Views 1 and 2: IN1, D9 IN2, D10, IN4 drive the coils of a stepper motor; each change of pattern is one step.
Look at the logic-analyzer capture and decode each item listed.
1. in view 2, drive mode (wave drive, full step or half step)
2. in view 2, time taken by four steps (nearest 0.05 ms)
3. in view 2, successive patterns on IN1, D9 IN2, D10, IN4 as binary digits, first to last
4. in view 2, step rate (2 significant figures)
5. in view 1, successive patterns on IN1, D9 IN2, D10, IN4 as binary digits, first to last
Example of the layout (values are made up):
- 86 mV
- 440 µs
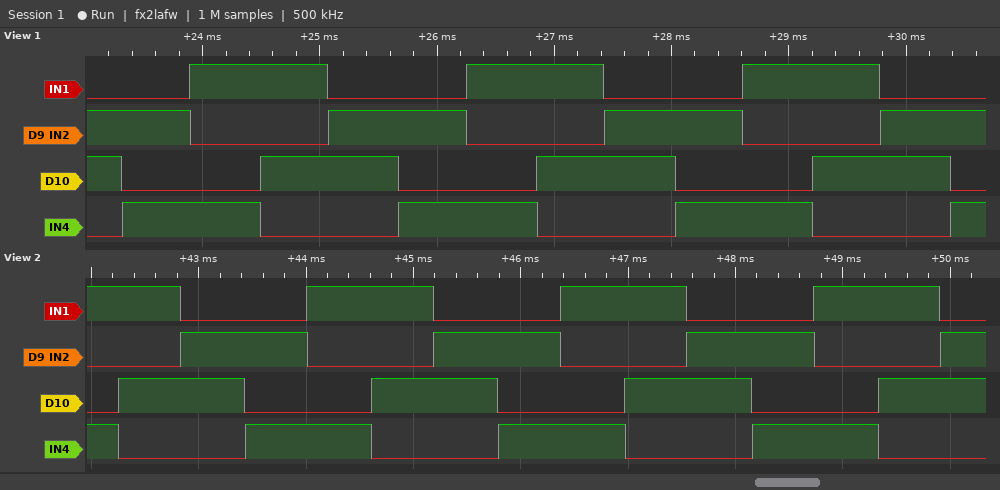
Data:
- full step
- 2.35 ms
- 1001 1010 0110 0101 1001 1010 0110 0101 1001 1010 0110 0101 1001 1010 0110
- 1700 steps/s
- 0110 0101 1001 1010 0110 0101 1001 1010 0110 0101 1001 1010 0110 0101
